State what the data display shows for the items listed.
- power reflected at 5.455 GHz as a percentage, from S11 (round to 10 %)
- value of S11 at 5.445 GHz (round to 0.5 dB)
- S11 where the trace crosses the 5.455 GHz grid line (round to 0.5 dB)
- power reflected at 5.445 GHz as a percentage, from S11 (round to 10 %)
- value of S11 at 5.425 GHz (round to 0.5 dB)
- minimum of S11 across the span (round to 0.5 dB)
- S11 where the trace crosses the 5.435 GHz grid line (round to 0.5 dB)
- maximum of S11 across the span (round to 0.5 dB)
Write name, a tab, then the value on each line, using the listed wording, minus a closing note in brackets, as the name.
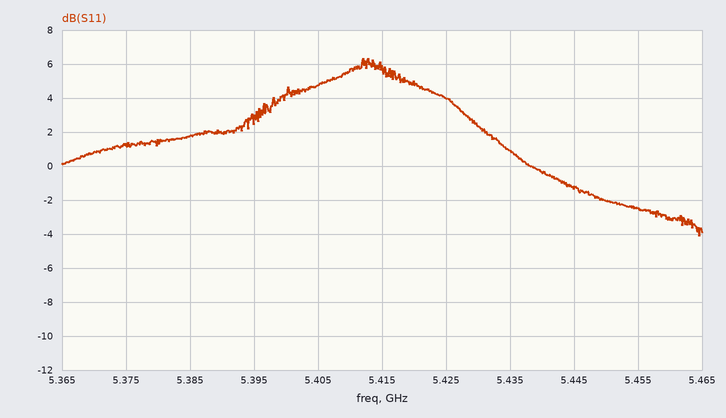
power reflected at 5.455 GHz as a percentage, from S11	60 %
value of S11 at 5.445 GHz	-1.5 dB
S11 where the trace crosses the 5.455 GHz grid line	-2.5 dB
power reflected at 5.445 GHz as a percentage, from S11	70 %
value of S11 at 5.425 GHz	4.0 dB
minimum of S11 across the span	-4.0 dB
S11 where the trace crosses the 5.435 GHz grid line	1.0 dB
maximum of S11 across the span	6.5 dB
